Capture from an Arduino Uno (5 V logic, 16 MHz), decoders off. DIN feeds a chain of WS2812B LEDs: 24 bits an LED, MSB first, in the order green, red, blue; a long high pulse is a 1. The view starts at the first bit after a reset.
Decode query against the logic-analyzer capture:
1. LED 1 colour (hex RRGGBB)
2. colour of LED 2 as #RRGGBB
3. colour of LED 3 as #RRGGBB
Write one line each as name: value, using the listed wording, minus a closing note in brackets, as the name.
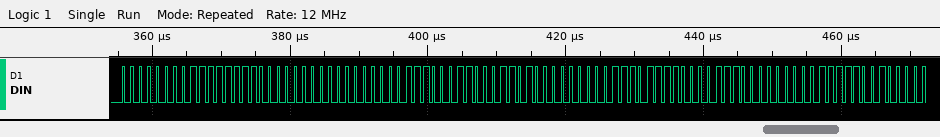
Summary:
LED 1 colour: #FF0000
colour of LED 2 as #RRGGBB: #71008D
colour of LED 3 as #RRGGBB: #770087
